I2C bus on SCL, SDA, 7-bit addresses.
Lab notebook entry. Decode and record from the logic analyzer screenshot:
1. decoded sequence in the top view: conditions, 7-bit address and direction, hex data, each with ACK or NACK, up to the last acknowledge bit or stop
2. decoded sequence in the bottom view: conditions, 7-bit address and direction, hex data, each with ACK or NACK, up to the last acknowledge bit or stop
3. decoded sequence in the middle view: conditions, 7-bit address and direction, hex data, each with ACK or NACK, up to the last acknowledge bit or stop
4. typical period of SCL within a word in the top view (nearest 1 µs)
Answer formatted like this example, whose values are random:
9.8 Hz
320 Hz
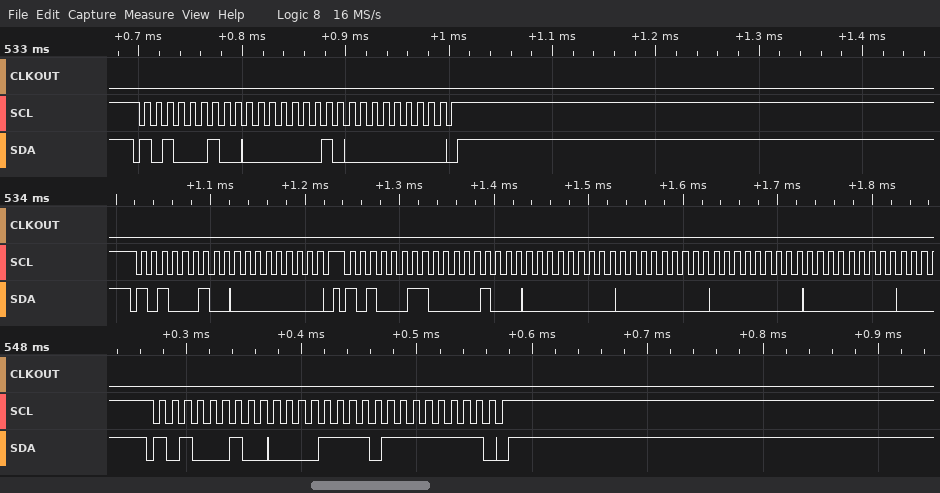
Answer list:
start, address 51 write ACK, 01 ACK, 00 ACK, stop
start, address 51 write ACK, 0F ACK, FF ACK, stop
start, address 51 write ACK, 00 ACK, stop, start, address 51 read ACK, 08 ACK, 00 ACK, 00 ACK, 00 ACK, 00 ACK
11 µs
